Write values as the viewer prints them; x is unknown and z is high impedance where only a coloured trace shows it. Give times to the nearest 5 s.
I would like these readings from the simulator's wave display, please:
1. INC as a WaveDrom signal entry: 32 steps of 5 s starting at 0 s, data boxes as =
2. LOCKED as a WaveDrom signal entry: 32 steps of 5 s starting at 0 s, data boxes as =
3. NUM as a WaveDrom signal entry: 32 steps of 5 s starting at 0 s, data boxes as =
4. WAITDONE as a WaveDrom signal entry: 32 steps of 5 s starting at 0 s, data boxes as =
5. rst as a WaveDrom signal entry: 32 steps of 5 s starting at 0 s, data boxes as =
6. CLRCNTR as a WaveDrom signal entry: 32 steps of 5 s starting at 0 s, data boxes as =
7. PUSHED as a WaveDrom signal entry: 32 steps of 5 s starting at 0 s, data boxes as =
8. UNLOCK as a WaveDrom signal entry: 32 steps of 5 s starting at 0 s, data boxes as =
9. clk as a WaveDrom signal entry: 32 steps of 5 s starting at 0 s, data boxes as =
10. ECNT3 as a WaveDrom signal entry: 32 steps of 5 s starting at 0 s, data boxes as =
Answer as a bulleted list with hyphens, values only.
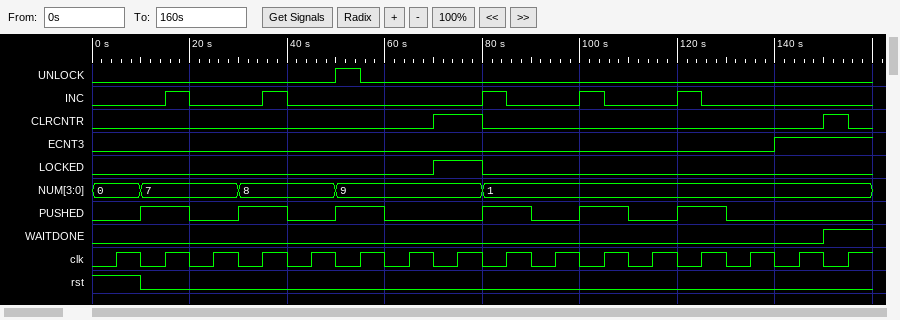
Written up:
- {name: 'INC', wave: '0..10..10.......10..10..10......'}
- {name: 'LOCKED', wave: '0.............1.0...............'}
- {name: 'NUM', wave: '=.=...=...=.....=...............', data: '0 7 8 9 1'}
- {name: 'WAITDONE', wave: '0.............................1.'}
- {name: 'rst', wave: '1.0.............................'}
- {name: 'CLRCNTR', wave: '0.............1.0.............10'}
- {name: 'PUSHED', wave: '0.1.0.1.0.1.0...1.0.1.0.1.0.....'}
- {name: 'UNLOCK', wave: '0.........10....................'}
- {name: 'clk', wave: '01010101010101010101010101010101'}
- {name: 'ECNT3', wave: '0...........................1...'}
